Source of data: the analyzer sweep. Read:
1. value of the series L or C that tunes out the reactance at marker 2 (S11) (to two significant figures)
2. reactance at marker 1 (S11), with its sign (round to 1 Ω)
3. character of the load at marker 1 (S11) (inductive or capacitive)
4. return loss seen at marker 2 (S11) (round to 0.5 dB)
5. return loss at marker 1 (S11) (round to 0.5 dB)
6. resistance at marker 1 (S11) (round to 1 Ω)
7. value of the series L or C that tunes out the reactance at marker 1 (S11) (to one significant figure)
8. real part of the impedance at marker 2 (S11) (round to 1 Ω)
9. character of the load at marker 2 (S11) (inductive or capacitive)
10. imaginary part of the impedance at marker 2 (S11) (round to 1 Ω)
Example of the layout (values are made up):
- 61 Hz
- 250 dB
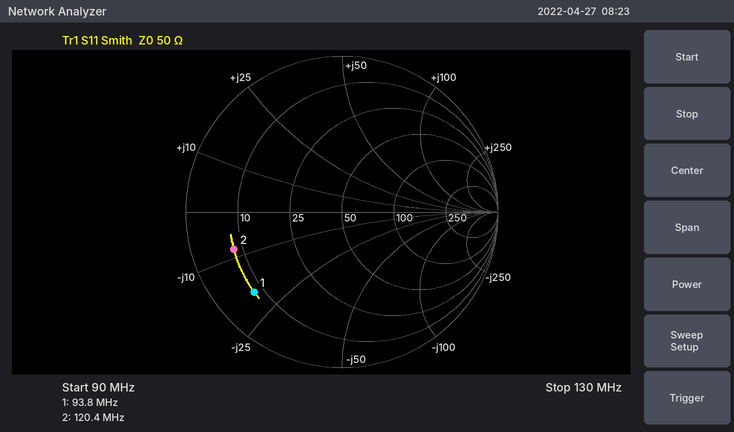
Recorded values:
- 11 nH
- -19 Ω
- capacitive
- 2.5 dB
- 2.5 dB
- 8 Ω
- 30 nH
- 8 Ω
- capacitive
- -8 Ω
